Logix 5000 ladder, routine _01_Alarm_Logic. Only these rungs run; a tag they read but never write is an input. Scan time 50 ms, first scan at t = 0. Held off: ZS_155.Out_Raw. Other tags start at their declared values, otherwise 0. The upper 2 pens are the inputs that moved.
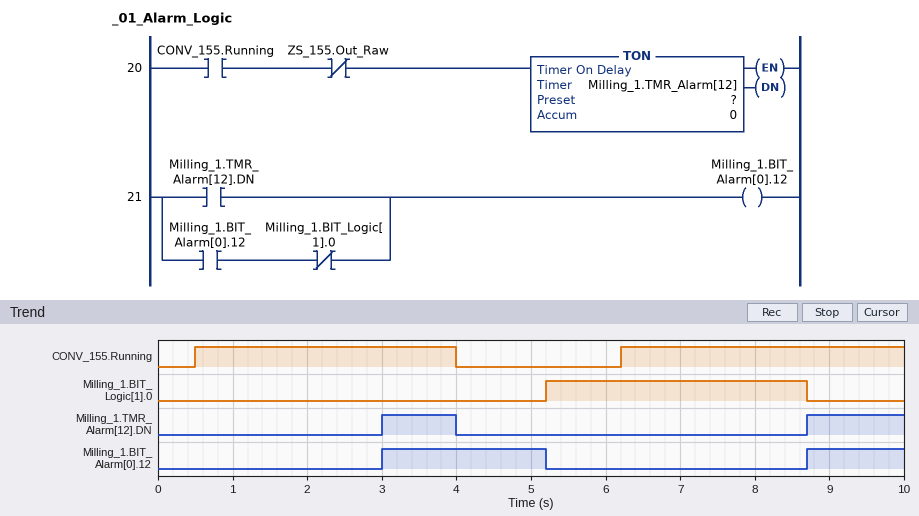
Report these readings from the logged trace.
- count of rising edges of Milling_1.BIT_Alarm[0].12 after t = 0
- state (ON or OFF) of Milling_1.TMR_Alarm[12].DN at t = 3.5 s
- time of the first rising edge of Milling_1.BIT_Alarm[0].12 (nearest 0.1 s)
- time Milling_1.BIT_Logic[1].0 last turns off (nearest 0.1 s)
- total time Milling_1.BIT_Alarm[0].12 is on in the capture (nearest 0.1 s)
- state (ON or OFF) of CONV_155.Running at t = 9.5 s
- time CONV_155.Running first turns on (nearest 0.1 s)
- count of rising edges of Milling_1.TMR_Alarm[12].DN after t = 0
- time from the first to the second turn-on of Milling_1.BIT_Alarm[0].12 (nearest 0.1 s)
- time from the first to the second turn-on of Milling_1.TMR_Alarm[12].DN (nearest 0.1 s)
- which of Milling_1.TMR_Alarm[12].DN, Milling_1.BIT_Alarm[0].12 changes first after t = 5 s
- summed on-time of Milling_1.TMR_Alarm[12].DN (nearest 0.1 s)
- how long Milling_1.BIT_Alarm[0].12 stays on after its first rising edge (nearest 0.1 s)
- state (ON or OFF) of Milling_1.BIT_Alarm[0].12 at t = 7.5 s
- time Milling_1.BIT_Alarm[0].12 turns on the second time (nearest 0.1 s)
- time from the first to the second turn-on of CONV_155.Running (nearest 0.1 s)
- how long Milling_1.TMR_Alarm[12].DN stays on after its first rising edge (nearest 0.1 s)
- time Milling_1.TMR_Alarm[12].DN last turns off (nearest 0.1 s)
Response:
2
ON
3.0 s
8.7 s
3.5 s
ON
0.5 s
2
5.7 s
5.7 s
Milling_1.BIT_Alarm[0].12
2.3 s
2.2 s
OFF
8.7 s
5.7 s
1.0 s
4.0 s
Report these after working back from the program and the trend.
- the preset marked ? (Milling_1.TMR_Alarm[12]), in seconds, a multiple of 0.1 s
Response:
2.5 s
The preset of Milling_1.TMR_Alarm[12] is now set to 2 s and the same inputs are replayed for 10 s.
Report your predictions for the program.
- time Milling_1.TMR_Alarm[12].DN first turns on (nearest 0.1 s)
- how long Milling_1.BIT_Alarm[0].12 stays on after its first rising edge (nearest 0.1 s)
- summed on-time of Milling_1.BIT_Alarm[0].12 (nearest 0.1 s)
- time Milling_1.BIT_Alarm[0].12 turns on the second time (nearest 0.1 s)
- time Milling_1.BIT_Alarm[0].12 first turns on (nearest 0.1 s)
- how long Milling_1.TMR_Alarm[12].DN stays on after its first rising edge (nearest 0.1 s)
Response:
2.5 s
2.7 s
4.5 s
8.2 s
2.5 s
1.5 s
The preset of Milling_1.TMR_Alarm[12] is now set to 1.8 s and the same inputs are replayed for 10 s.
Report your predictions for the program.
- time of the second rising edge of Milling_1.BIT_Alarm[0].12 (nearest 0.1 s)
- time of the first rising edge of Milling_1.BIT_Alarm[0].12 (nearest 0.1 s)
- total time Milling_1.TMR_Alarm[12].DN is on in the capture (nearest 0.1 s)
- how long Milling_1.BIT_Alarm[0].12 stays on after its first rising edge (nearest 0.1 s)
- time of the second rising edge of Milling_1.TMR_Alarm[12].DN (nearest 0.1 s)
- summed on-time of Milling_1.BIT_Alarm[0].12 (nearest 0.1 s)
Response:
8.0 s
2.3 s
3.7 s
2.9 s
8.0 s
4.9 s
